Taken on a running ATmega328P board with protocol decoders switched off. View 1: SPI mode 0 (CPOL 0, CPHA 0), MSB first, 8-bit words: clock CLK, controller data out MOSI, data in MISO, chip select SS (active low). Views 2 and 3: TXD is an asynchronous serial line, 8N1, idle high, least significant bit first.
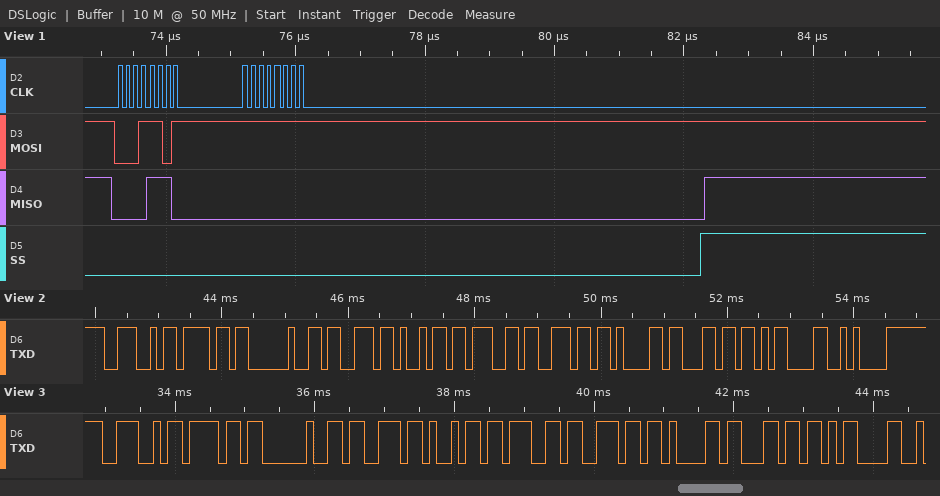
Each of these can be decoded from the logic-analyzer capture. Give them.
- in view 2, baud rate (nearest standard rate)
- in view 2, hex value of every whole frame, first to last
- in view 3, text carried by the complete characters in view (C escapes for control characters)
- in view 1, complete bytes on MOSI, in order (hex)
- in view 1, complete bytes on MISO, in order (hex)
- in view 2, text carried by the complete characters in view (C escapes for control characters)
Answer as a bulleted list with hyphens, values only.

- 9600 baud
- 4E 6F 20 73 69 67 6E 61 6C 0D 0A
- "No signal\r"
- 1D FF
- 0E 00
- "No signal\r\n"
